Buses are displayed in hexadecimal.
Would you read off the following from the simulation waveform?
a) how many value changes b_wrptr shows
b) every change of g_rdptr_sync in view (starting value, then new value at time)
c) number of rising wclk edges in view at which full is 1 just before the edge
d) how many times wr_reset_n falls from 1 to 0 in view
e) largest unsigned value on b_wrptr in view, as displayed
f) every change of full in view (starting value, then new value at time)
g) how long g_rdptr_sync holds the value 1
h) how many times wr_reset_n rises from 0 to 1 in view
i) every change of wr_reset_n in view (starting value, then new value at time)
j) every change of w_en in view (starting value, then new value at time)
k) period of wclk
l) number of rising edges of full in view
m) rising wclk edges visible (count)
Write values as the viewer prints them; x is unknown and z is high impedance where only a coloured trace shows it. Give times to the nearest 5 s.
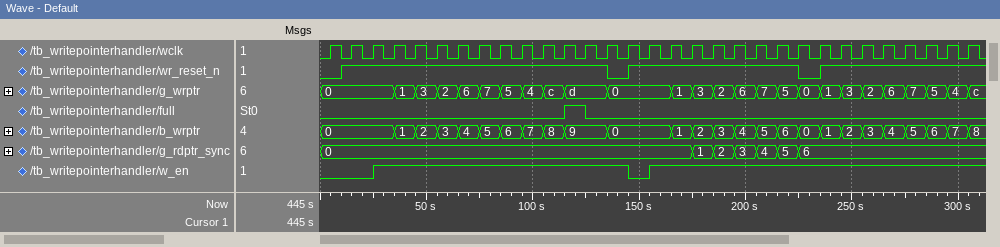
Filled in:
25
0, 1 at 175 s, 2 at 185 s, 3 at 195 s, 4 at 205 s, 5 at 215 s, 6 at 225 s
1
2
9
0, 1 at 115 s, 0 at 125 s
10 s
3
0, 1 at 10 s, 0 at 135 s, 1 at 145 s, 0 at 225 s, 1 at 235 s
0, 1 at 25 s, 0 at 145 s, 1 at 155 s
10 s
1
31
